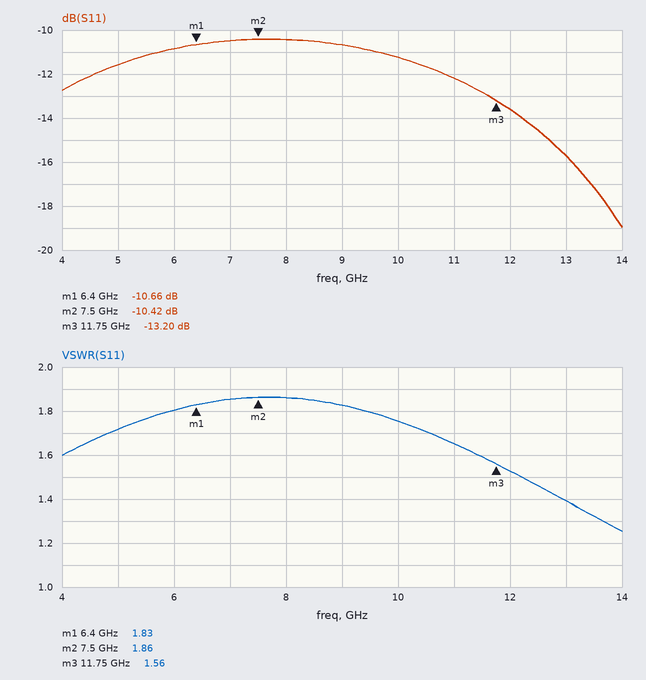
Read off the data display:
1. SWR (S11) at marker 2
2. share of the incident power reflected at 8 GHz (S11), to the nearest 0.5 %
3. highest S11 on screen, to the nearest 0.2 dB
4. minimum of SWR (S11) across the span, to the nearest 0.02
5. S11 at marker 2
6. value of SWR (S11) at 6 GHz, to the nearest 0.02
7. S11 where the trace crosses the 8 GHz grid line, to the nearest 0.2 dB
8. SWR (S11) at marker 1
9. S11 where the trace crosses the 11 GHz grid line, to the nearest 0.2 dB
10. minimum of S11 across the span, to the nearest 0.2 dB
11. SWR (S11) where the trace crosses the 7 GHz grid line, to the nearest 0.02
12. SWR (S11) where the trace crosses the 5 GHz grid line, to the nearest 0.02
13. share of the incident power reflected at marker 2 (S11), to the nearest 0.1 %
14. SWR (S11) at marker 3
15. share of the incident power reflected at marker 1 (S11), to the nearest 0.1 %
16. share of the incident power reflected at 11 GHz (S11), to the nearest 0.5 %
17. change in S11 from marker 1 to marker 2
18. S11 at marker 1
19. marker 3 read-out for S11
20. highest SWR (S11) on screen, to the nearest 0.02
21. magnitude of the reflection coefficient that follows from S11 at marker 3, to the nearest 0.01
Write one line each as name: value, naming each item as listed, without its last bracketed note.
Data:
SWR (S11) at marker 2: 1.86
share of the incident power reflected at 8 GHz (S11), to the nearest 0.5 %: 9.0 %
highest S11 on screen, to the nearest 0.2 dB: -10.4 dB
minimum of SWR (S11) across the span, to the nearest 0.02: 1.26
S11 at marker 2: -10.42 dB
value of SWR (S11) at 6 GHz, to the nearest 0.02: 1.80
S11 where the trace crosses the 8 GHz grid line, to the nearest 0.2 dB: -10.4 dB
SWR (S11) at marker 1: 1.83
S11 where the trace crosses the 11 GHz grid line, to the nearest 0.2 dB: -12.2 dB
minimum of S11 across the span, to the nearest 0.2 dB: -19.0 dB
SWR (S11) where the trace crosses the 7 GHz grid line, to the nearest 0.02: 1.86
SWR (S11) where the trace crosses the 5 GHz grid line, to the nearest 0.02: 1.72
share of the incident power reflected at marker 2 (S11), to the nearest 0.1 %: 9.1 %
SWR (S11) at marker 3: 1.56
share of the incident power reflected at marker 1 (S11), to the nearest 0.1 %: 8.6 %
share of the incident power reflected at 11 GHz (S11), to the nearest 0.5 %: 6.0 %
change in S11 from marker 1 to marker 2: 0.24 dB
S11 at marker 1: -10.66 dB
marker 3 read-out for S11: -13.20 dB
highest SWR (S11) on screen, to the nearest 0.02: 1.86
magnitude of the reflection coefficient that follows from S11 at marker 3, to the nearest 0.01: 0.22
